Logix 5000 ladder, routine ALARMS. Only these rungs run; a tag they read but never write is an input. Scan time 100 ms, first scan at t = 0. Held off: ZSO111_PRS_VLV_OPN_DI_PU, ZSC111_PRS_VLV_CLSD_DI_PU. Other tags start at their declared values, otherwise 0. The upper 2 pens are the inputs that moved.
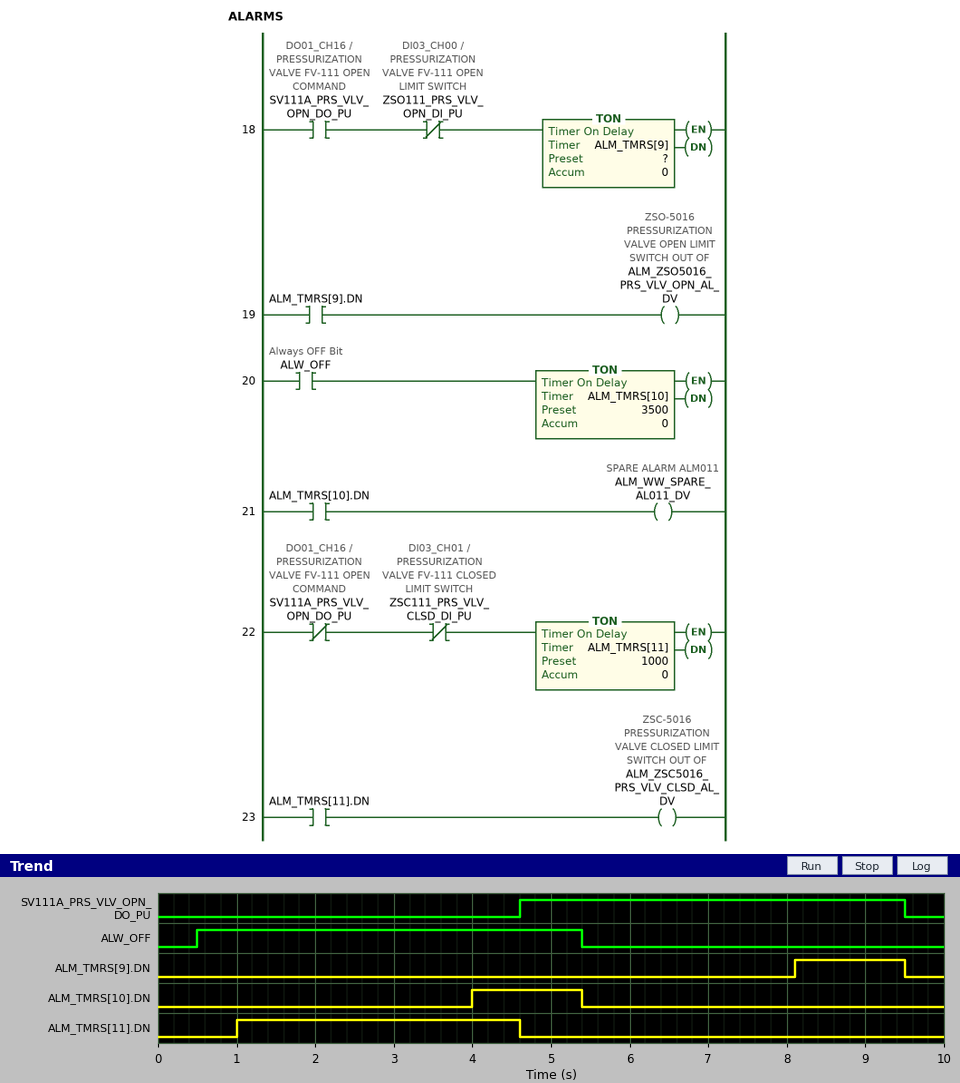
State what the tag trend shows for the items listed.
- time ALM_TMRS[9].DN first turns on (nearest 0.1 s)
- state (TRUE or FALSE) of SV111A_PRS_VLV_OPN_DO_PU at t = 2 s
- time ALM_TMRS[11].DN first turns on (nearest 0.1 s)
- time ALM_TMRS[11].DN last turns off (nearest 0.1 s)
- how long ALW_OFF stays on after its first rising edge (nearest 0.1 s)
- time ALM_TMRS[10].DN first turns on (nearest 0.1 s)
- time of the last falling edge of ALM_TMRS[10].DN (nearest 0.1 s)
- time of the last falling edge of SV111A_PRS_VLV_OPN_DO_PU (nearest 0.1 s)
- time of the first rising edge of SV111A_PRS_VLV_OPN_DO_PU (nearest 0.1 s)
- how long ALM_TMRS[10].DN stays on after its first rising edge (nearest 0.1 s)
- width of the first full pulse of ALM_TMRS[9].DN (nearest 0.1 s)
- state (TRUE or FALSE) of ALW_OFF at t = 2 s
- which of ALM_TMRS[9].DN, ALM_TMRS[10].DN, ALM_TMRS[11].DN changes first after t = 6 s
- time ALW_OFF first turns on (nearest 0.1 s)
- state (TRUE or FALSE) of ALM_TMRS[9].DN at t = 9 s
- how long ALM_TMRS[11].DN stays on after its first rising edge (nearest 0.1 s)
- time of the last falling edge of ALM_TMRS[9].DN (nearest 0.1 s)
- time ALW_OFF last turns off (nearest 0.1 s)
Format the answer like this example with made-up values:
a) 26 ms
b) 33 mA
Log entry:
a) 8.1 s
b) FALSE
c) 1.0 s
d) 4.6 s
e) 4.9 s
f) 4.0 s
g) 5.4 s
h) 9.5 s
i) 4.6 s
j) 1.4 s
k) 1.4 s
l) TRUE
m) ALM_TMRS[9].DN
n) 0.5 s
o) TRUE
p) 3.6 s
q) 9.5 s
r) 5.4 s
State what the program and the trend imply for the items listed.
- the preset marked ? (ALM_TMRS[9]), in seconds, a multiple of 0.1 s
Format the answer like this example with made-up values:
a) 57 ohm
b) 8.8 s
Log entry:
a) 3.5 s
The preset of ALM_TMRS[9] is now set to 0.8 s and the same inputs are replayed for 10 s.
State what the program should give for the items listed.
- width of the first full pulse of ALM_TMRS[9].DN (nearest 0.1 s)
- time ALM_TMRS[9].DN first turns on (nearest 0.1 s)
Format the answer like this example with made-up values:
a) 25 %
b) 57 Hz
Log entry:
a) 4.1 s
b) 5.4 s
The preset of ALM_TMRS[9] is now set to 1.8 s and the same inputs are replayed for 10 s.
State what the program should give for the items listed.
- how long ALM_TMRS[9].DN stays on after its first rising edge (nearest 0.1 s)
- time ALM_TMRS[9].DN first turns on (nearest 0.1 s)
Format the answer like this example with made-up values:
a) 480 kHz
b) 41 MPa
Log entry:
a) 3.1 s
b) 6.4 s
